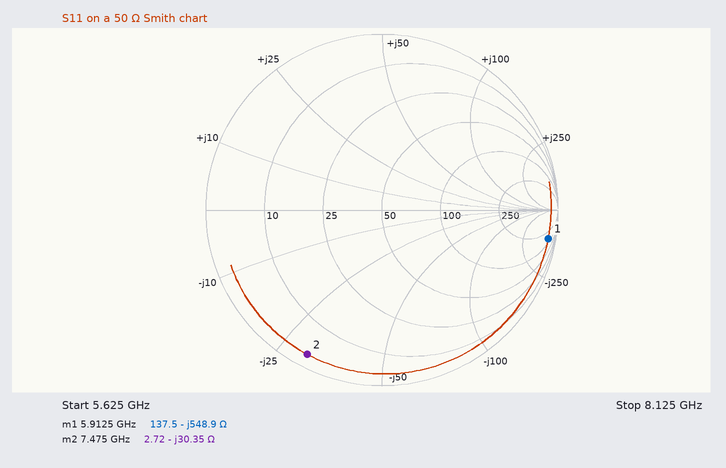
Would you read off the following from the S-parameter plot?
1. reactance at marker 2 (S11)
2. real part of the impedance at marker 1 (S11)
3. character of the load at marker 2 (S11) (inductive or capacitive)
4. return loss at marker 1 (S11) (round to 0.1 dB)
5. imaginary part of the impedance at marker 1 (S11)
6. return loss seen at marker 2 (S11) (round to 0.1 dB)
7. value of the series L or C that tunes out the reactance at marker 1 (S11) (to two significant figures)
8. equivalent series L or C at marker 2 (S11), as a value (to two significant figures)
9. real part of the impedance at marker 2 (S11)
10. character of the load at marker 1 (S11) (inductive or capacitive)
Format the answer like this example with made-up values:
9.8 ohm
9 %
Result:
-30.35 Ω
137.5 Ω
capacitive
0.4 dB
-548.9 Ω
0.7 dB
15 nH
700 fF
2.72 Ω
capacitive
